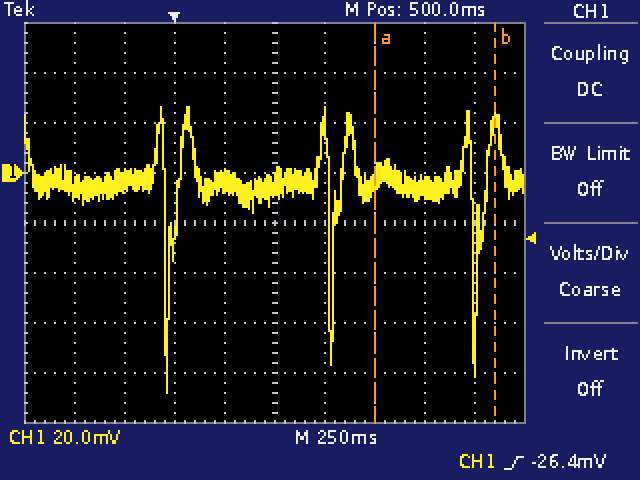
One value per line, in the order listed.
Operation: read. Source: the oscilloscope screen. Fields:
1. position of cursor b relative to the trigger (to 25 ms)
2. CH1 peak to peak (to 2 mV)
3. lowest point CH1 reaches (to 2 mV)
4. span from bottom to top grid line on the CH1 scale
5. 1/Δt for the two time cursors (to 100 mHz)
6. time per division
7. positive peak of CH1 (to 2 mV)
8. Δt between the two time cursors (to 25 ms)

+1.600 s
114 mV
-88 mV
160 mV
1.7 Hz
250 ms
26 mV
600 ms
